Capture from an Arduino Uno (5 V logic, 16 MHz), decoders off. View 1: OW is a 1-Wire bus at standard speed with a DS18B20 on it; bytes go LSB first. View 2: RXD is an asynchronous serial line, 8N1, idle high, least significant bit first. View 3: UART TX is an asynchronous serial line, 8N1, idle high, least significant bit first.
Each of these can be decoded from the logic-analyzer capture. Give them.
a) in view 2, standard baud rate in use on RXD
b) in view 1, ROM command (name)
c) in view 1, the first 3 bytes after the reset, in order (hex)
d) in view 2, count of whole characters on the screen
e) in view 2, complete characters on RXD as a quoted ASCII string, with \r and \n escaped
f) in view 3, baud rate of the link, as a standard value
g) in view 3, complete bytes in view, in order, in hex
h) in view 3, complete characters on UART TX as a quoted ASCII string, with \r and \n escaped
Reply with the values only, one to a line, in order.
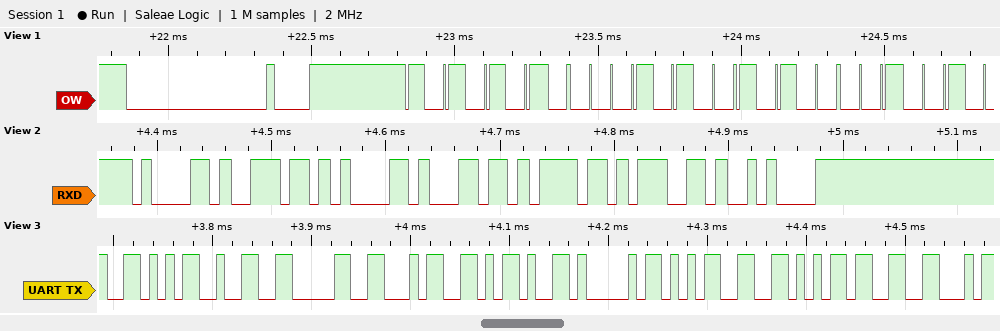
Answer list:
115200 baud
Match ROM
55 28 85
7
"analog\n"
115200 baud
56 32 30 34 2D 41 35 56 33
"V204-A5V3"
